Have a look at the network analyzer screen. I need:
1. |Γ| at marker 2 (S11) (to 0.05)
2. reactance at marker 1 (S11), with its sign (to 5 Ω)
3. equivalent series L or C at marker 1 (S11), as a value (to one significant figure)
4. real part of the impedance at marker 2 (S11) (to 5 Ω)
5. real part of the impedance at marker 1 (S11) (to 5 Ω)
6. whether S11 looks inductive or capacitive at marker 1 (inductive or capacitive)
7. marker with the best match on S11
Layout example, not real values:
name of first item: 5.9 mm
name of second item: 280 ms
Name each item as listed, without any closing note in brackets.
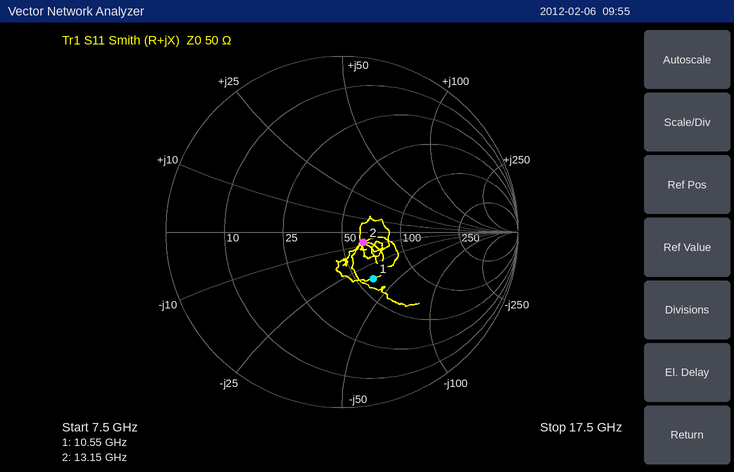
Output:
|Γ| at marker 2 (S11): 0.15
reactance at marker 1 (S11), with its sign: -35 Ω
equivalent series L or C at marker 1 (S11), as a value: 400 fF
real part of the impedance at marker 2 (S11): 65 Ω
real part of the impedance at marker 1 (S11): 60 Ω
whether S11 looks inductive or capacitive at marker 1: capacitive
marker with the best match on S11: marker 2
